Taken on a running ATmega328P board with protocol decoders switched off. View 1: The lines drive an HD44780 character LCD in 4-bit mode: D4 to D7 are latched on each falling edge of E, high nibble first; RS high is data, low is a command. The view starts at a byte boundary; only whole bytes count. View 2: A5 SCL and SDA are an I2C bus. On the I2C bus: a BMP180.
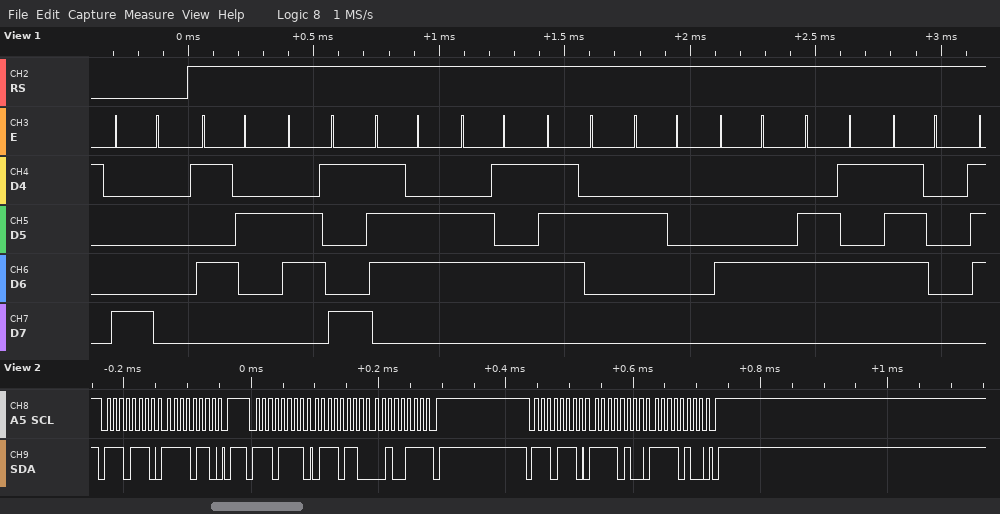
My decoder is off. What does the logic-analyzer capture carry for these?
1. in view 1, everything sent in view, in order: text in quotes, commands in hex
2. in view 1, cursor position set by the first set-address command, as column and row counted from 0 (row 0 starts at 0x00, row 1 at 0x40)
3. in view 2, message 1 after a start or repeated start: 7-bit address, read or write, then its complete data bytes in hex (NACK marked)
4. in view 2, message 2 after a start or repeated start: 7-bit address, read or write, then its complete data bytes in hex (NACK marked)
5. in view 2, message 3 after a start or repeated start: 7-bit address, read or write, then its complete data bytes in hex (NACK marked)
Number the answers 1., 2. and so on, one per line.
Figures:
1. 0x80 "River Dep"
2. column 0, row 0
3. 0x77 write: F6
4. 0x77 read: 76 27 NACK
5. 0x77 write: F4 F4
